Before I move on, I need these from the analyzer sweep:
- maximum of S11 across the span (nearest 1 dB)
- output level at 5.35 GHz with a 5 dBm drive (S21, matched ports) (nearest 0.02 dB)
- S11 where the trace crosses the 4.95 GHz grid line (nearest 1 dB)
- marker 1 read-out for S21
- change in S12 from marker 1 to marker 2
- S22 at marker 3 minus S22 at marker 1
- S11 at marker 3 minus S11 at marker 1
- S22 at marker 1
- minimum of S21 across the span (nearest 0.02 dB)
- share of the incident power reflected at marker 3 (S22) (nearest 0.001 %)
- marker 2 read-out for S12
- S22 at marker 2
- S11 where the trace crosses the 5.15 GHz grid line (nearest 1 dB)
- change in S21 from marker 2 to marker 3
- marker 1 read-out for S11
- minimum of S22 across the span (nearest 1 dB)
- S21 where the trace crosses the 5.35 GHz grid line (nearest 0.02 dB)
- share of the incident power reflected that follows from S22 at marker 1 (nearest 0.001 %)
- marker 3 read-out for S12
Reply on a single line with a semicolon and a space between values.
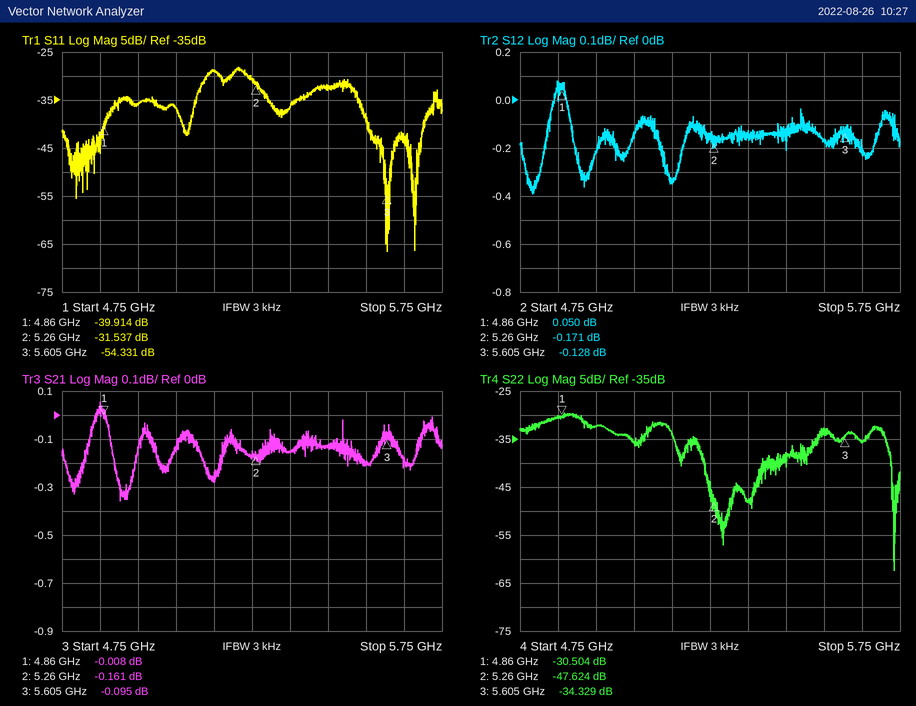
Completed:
-28 dB; 4.84 dBm; -36 dB; -0.008 dB; -0.221 dB; -3.825 dB; -14.417 dB; -30.504 dB; -0.36 dB; 0.037 %; -0.171 dB; -47.624 dB; -29 dB; 0.066 dB; -39.914 dB; -62 dB; -0.16 dB; 0.089 %; -0.128 dB
